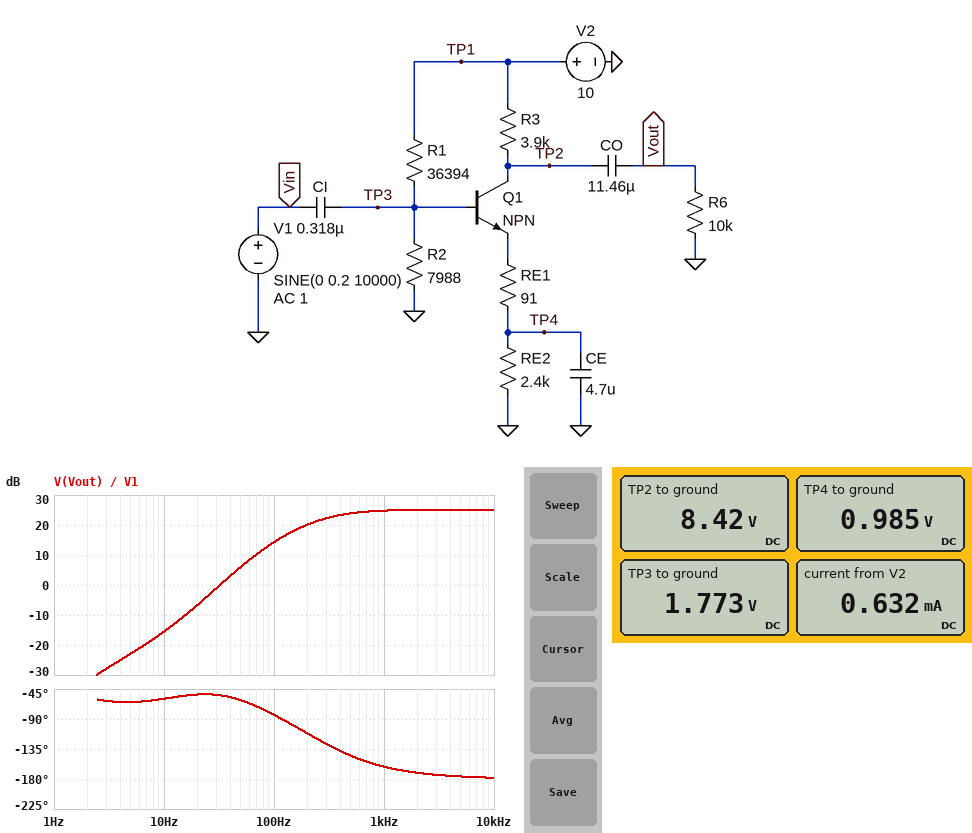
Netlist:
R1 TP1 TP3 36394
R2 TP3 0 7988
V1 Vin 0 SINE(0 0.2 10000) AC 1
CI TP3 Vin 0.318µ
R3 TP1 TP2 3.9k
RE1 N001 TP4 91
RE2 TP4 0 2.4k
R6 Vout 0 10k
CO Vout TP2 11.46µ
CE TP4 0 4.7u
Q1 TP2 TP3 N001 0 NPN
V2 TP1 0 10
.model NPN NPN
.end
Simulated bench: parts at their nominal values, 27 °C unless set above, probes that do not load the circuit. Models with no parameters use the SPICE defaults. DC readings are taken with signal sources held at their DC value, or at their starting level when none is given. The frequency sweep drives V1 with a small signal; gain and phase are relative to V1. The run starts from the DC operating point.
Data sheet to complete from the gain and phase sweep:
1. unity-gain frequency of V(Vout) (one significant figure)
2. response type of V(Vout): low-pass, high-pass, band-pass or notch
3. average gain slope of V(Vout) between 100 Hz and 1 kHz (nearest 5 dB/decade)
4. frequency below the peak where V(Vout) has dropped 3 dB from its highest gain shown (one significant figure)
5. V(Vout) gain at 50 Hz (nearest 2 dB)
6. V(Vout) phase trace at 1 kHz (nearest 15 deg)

30 Hz
high-pass
10 dB/decade
300 Hz
6 dB
-165 deg
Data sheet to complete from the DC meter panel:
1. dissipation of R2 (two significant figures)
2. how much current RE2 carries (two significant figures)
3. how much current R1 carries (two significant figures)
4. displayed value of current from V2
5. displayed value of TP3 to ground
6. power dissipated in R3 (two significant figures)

390 µW
410 µA
230 µA
0.632 mA
1.773 V
640 µW
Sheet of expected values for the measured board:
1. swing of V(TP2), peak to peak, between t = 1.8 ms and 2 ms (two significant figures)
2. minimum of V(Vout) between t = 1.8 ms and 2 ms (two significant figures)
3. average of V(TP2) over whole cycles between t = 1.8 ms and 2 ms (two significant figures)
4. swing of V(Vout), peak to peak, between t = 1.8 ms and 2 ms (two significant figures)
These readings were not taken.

4.3 V
-3.2 V
8.2 V
4.3 V
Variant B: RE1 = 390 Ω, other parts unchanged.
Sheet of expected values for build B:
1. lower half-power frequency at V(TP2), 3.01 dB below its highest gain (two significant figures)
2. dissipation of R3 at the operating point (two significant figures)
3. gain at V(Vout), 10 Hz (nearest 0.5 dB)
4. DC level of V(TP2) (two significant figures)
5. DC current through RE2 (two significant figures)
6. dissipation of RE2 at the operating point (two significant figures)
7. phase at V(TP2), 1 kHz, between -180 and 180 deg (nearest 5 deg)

140 Hz
520 µW
-16.5 dB
8.6 V
370 µA
330 µW
-170 deg
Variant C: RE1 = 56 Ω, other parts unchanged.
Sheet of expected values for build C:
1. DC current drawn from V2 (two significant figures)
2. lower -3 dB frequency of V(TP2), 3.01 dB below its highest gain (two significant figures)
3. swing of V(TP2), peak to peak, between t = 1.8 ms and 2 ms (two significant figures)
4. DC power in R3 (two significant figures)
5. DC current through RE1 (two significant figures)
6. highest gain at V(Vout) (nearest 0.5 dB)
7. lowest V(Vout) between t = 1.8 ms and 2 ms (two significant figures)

640 µA
360 Hz
5.0 V
660 µW
420 µA
27.5 dB
-3.9 V
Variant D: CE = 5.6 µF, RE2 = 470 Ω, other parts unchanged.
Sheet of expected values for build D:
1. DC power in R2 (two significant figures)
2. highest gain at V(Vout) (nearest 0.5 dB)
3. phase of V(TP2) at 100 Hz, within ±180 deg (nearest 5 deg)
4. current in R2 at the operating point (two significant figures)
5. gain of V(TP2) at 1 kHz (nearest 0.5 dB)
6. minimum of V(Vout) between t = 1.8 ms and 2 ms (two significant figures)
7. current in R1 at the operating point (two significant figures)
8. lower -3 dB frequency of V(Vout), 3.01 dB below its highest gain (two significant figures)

360 µW
28.5 dB
-100 deg
210 µA
27.5 dB
-2.8 V
230 µA
380 Hz
